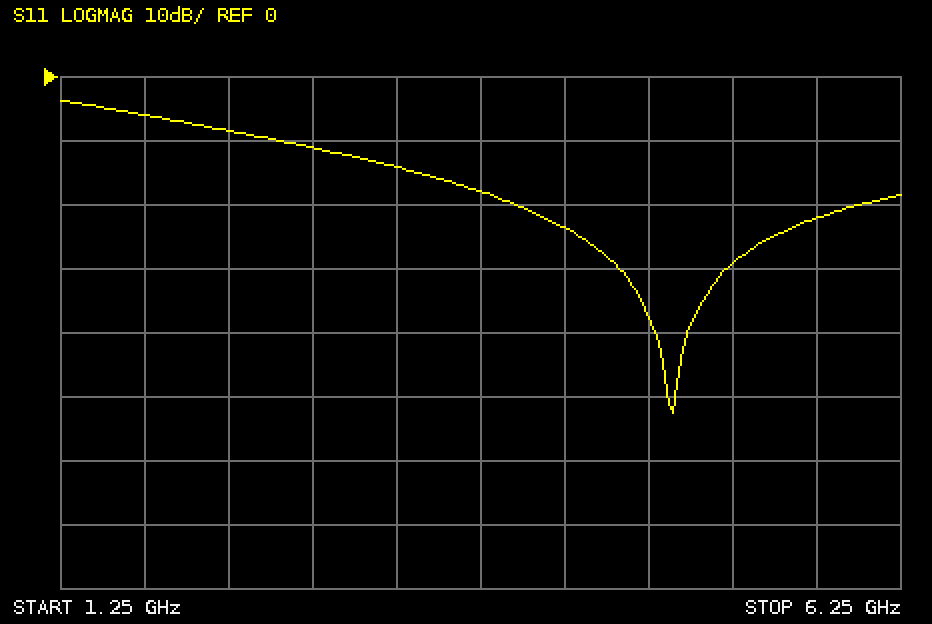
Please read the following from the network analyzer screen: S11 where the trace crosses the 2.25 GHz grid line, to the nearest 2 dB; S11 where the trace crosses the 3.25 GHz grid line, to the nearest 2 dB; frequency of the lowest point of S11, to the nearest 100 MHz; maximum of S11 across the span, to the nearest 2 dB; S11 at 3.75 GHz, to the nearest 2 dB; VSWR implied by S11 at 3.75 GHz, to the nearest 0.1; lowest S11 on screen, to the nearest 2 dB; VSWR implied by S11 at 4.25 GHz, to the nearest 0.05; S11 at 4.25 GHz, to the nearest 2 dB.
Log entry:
-8 dB
-14 dB
4.9 GHz
-4 dB
-18 dB
1.3
-52 dB
1.15
-24 dB
